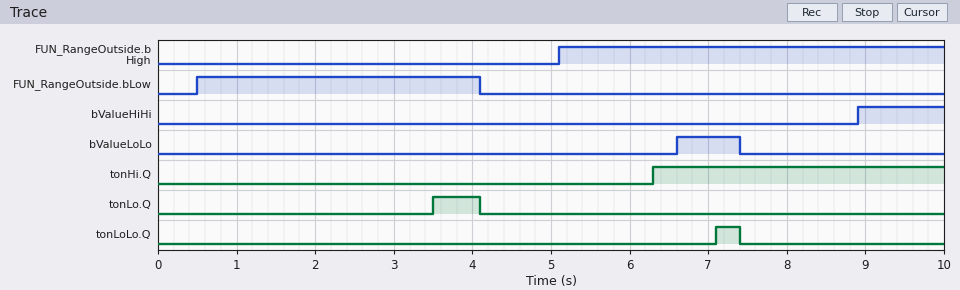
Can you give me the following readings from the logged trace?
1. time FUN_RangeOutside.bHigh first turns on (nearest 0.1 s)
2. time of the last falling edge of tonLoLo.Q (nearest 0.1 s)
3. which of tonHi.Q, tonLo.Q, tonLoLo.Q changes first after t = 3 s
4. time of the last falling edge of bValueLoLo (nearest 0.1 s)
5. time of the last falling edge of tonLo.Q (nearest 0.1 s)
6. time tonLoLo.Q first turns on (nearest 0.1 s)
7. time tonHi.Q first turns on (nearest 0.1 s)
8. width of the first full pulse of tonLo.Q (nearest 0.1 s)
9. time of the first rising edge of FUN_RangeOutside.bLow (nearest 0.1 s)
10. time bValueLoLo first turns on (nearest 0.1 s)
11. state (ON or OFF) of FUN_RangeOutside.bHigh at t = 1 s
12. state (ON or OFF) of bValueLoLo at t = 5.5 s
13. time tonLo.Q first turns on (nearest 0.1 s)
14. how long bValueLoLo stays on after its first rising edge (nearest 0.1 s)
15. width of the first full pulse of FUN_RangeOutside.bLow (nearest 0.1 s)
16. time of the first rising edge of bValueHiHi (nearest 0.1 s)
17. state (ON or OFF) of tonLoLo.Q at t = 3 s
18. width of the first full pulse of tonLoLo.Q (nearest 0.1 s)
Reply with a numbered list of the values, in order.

1. 5.1 s
2. 7.4 s
3. tonLo.Q
4. 7.4 s
5. 4.1 s
6. 7.1 s
7. 6.3 s
8. 0.6 s
9. 0.5 s
10. 6.6 s
11. OFF
12. OFF
13. 3.5 s
14. 0.8 s
15. 3.6 s
16. 8.9 s
17. OFF
18. 0.3 s
